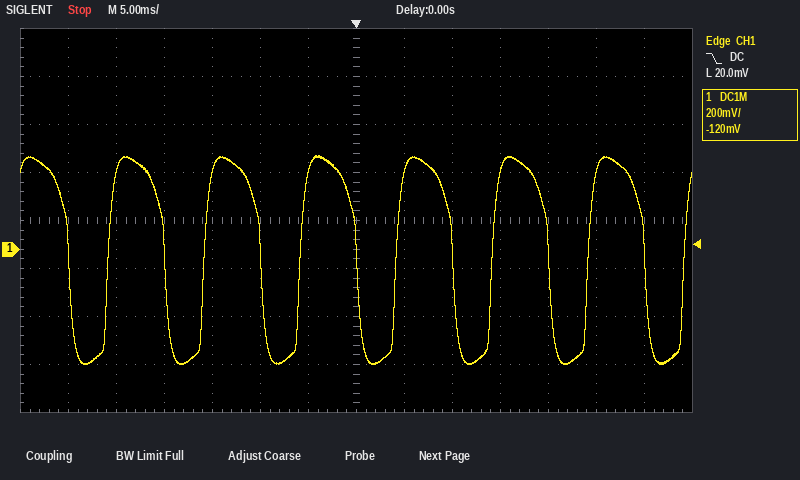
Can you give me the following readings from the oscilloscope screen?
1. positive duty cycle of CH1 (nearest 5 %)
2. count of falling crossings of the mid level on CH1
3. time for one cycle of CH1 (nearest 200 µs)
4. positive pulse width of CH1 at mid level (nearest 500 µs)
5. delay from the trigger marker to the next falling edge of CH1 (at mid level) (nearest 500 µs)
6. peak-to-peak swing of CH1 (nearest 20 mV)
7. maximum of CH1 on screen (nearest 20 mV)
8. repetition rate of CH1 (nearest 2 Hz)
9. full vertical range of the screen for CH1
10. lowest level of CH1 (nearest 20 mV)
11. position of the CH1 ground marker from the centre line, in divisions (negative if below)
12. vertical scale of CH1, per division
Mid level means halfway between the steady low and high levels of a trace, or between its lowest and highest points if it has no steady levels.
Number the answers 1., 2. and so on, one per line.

1. 60 %
2. 7
3. 10.0 ms
4. 6.0 ms
5. 10.0 ms
6. 880 mV
7. 400 mV
8. 100 Hz
9. 1.6 V
10. -480 mV
11. -0.6 div
12. 200 mV
